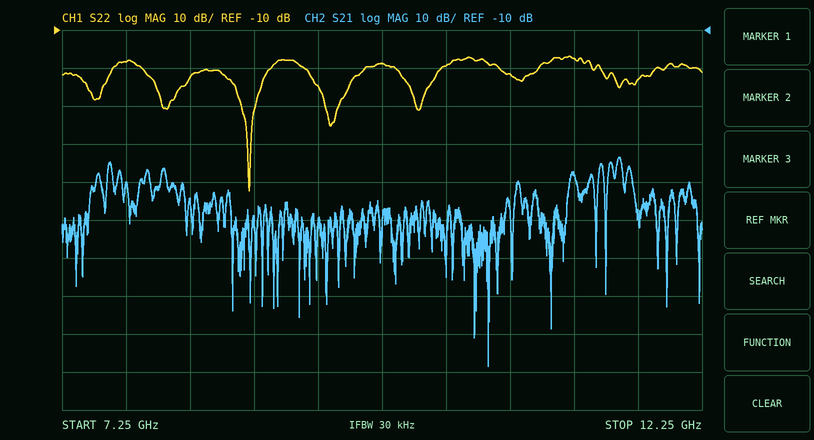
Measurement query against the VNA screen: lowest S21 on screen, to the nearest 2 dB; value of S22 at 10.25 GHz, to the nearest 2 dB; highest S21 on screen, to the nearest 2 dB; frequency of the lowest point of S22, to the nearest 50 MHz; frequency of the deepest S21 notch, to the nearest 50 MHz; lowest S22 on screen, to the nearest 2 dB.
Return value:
-98 dB
-20 dB
-44 dB
8.70 GHz
10.60 GHz
-52 dB
